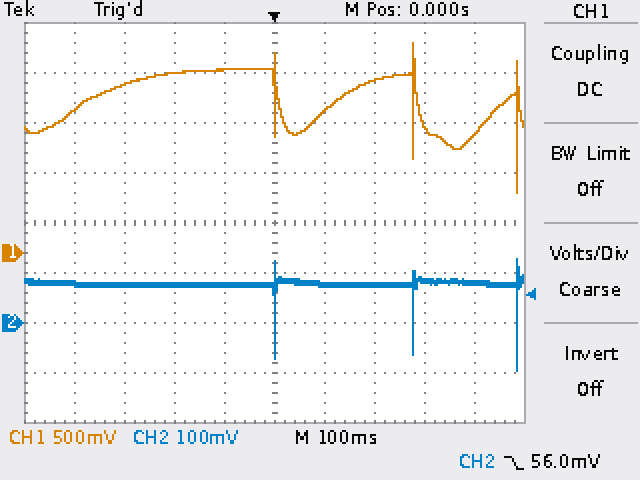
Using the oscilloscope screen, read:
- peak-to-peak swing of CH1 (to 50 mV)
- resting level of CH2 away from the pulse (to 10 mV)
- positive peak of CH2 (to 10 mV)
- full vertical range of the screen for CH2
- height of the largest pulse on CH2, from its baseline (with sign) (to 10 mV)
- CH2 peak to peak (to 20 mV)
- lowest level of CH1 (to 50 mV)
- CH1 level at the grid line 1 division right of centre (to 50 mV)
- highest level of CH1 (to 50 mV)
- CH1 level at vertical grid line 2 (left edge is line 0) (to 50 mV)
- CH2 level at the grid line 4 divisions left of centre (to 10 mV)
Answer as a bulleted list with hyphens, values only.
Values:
- 1.50 V
- 80 mV
- 130 mV
- 800 mV
- -170 mV
- 220 mV
- 600 mV
- 1.40 V
- 2.10 V
- 1.70 V
- 80 mV
